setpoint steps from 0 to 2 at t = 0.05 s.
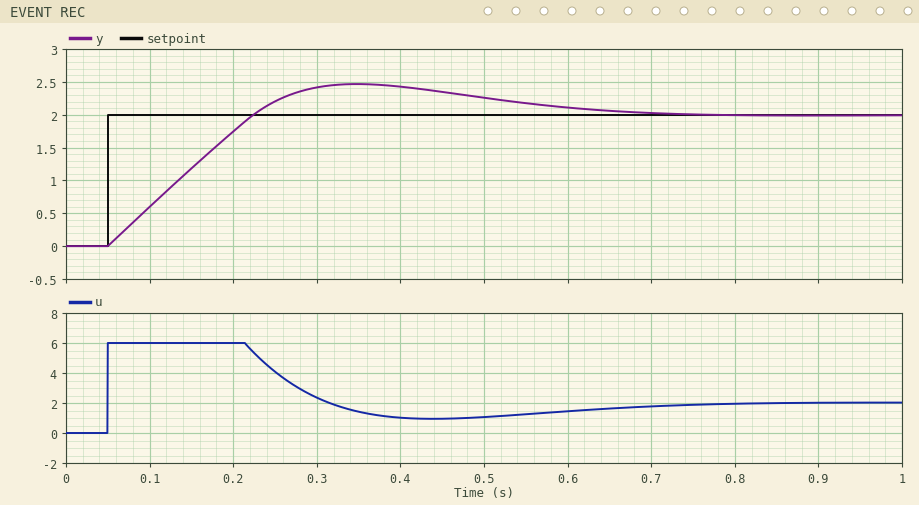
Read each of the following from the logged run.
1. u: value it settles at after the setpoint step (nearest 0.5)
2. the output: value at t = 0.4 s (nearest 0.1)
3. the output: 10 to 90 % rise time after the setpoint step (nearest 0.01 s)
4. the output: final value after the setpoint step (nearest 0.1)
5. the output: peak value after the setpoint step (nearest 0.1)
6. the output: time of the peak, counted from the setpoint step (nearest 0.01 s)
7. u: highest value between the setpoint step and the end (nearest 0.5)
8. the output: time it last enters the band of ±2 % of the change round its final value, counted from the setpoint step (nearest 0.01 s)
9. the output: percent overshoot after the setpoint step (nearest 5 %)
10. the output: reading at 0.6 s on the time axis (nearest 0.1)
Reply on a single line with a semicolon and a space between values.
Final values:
2.0; 2.4; 0.14 s; 2.0; 2.5; 0.30 s; 6.0; 0.63 s; 25 %; 2.1
